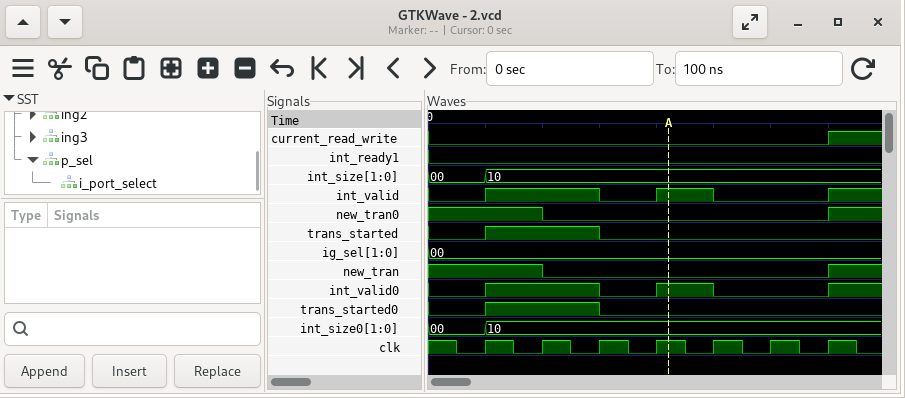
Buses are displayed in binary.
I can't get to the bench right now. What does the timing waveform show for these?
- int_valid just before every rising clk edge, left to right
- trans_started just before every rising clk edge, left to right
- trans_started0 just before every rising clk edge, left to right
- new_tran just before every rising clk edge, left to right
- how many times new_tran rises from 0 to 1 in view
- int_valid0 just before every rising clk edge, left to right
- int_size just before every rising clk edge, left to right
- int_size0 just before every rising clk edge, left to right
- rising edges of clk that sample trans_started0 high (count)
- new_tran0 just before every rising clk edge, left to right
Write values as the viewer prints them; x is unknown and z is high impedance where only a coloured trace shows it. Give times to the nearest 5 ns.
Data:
0 1 1 0 1 0 0
0 1 1 0 0 0 0
0 1 1 0 0 0 0
1 1 0 0 0 0 0
1
0 1 1 0 1 0 0
00, 10, 10, 10, 10, 10, 10
00, 10, 10, 10, 10, 10, 10
2
1 1 0 0 0 0 0
